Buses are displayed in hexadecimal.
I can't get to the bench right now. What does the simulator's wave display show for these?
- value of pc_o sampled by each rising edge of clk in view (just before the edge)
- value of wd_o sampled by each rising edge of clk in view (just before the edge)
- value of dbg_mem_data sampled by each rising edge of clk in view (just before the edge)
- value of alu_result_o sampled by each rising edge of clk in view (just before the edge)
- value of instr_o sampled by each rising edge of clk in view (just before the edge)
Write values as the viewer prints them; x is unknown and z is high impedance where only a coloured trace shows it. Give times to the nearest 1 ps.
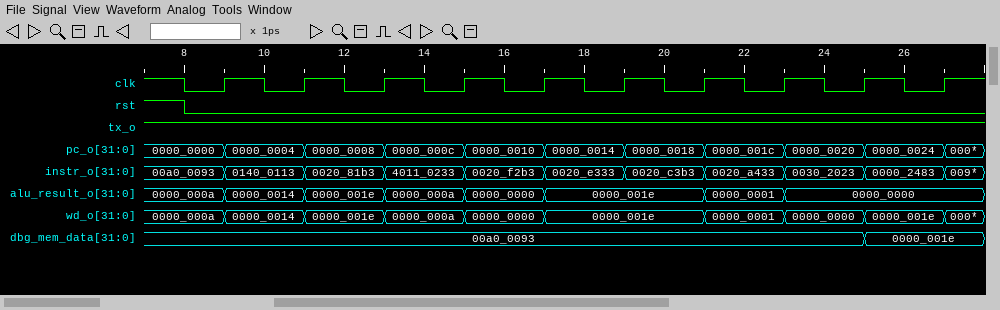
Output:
0000_0000, 0000_0004, 0000_0008, 0000_000c, 0000_0010, 0000_0014, 0000_0018, 0000_001c, 0000_0020, 0000_0024
0000_000a, 0000_0014, 0000_001e, 0000_000a, 0000_0000, 0000_001e, 0000_001e, 0000_0001, 0000_0000, 0000_001e
00a0_0093, 00a0_0093, 00a0_0093, 00a0_0093, 00a0_0093, 00a0_0093, 00a0_0093, 00a0_0093, 00a0_0093, 0000_001e
0000_000a, 0000_0014, 0000_001e, 0000_000a, 0000_0000, 0000_001e, 0000_001e, 0000_0001, 0000_0000, 0000_0000
00a0_0093, 0140_0113, 0020_81b3, 4011_0233, 0020_f2b3, 0020_e333, 0020_c3b3, 0020_a433, 0030_2023, 0000_2483
